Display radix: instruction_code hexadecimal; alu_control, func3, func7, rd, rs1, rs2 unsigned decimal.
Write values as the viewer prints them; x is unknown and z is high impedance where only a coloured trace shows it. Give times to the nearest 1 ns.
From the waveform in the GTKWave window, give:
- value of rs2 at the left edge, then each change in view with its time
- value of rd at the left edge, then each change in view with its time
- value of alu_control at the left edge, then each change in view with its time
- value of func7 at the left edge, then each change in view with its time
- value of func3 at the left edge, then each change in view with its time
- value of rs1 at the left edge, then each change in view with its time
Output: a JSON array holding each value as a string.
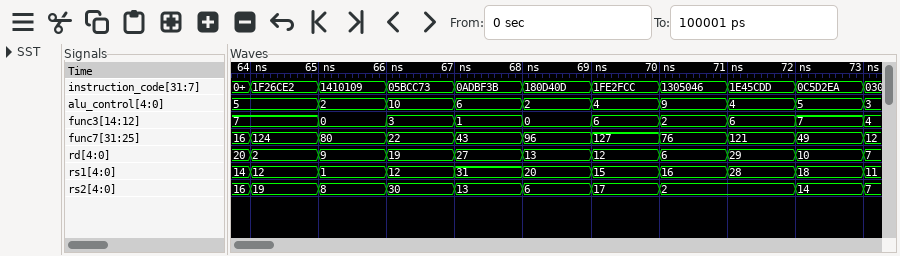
["16, 19 at 64 ns, 8 at 65 ns, 30 at 66 ns, 13 at 67 ns, 6 at 68 ns, 17 at 69 ns, 2 at 70 ns, 14 at 72 ns, 7 at 73 ns", "20, 2 at 64 ns, 9 at 65 ns, 19 at 66 ns, 27 at 67 ns, 13 at 68 ns, 12 at 69 ns, 6 at 70 ns, 29 at 71 ns, 10 at 72 ns, 7 at 73 ns", "5, 2 at 65 ns, 10 at 66 ns, 6 at 67 ns, 2 at 68 ns, 4 at 69 ns, 9 at 70 ns, 4 at 71 ns, 5 at 72 ns, 3 at 73 ns", "16, 124 at 64 ns, 80 at 65 ns, 22 at 66 ns, 43 at 67 ns, 96 at 68 ns, 127 at 69 ns, 76 at 70 ns, 121 at 71 ns, 49 at 72 ns, 12 at 73 ns", "7, 0 at 65 ns, 3 at 66 ns, 1 at 67 ns, 0 at 68 ns, 6 at 69 ns, 2 at 70 ns, 6 at 71 ns, 7 at 72 ns, 4 at 73 ns", "14, 12 at 64 ns, 1 at 65 ns, 12 at 66 ns, 31 at 67 ns, 20 at 68 ns, 15 at 69 ns, 16 at 70 ns, 28 at 71 ns, 18 at 72 ns, 11 at 73 ns"]
